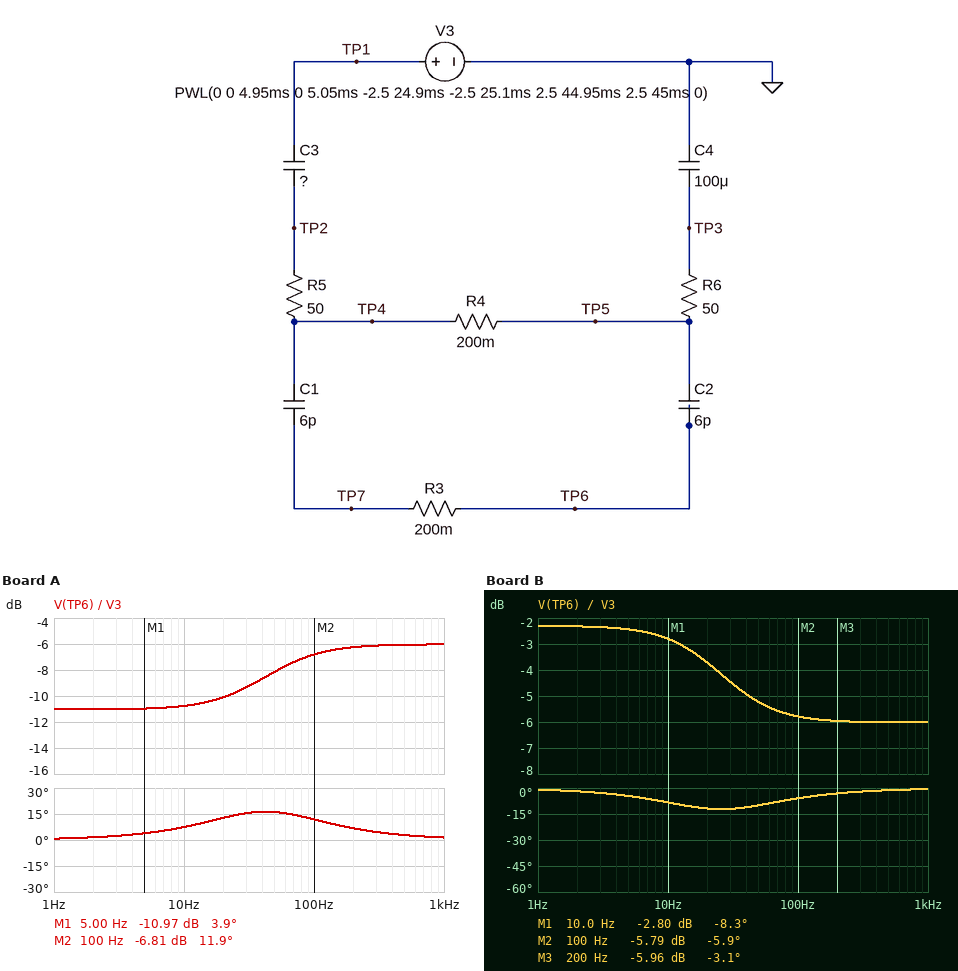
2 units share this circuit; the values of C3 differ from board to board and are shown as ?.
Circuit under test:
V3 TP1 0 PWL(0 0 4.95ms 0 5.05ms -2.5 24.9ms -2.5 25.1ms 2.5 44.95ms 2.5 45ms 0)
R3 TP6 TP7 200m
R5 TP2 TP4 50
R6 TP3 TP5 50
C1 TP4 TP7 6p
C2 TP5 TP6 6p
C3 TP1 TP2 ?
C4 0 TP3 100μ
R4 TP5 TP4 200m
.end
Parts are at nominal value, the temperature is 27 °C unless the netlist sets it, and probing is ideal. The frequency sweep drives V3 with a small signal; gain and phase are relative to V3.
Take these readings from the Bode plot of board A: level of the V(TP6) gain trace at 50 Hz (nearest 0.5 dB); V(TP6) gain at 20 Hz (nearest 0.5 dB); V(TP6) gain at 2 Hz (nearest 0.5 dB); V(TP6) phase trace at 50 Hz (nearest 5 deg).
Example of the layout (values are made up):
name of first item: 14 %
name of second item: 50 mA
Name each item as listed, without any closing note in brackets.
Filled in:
level of the V(TP6) gain trace at 50 Hz: -8.0 dB
V(TP6) gain at 20 Hz: -10.0 dB
V(TP6) gain at 2 Hz: -11.0 dB
V(TP6) phase trace at 50 Hz: 15 deg
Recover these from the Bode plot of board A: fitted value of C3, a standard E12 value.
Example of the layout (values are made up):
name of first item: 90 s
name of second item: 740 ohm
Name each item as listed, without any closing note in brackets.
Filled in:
fitted value of C3, a standard E12 value: 39 µF
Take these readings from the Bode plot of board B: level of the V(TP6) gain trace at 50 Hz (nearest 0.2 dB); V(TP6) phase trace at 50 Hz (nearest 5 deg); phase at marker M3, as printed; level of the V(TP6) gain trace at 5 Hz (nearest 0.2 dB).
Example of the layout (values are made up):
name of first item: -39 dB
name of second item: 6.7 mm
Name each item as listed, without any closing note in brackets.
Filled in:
level of the V(TP6) gain trace at 50 Hz: -5.2 dB
V(TP6) phase trace at 50 Hz: -10 deg
phase at marker M3, as printed: -3.1 deg
level of the V(TP6) gain trace at 5 Hz: -2.4 dB
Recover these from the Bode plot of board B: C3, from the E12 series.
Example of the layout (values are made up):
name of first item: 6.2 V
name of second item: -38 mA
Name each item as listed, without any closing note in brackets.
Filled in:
C3, from the E12 series: 330 µF
